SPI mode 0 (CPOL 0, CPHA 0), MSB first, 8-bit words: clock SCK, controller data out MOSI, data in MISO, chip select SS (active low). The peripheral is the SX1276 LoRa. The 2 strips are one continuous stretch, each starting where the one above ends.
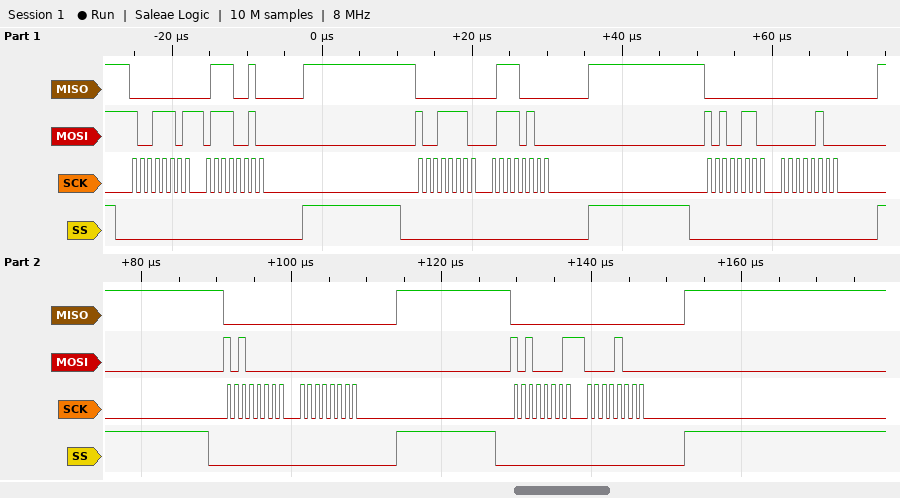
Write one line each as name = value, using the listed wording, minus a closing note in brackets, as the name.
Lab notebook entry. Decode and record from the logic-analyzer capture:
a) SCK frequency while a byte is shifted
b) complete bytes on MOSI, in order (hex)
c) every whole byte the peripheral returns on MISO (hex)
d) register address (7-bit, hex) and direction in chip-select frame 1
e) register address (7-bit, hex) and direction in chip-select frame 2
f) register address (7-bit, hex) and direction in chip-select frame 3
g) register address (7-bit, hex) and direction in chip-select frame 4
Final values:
SCK frequency while a byte is shifted = 1 MHz
complete bytes on MOSI, in order = 0x9D 0x72 0x9E 0x74 0xA6 0x04 0xA0 0x00 0xA1 0x08
every whole byte the peripheral returns on MISO = 0x00 0x72 0x00 0x70 0x00 0x00 0x00 0x00 0x00 0x00
register address (7-bit, hex) and direction in chip-select frame 1 = 0x1D write
register address (7-bit, hex) and direction in chip-select frame 2 = 0x1E write
register address (7-bit, hex) and direction in chip-select frame 3 = 0x26 write
register address (7-bit, hex) and direction in chip-select frame 4 = 0x20 write
